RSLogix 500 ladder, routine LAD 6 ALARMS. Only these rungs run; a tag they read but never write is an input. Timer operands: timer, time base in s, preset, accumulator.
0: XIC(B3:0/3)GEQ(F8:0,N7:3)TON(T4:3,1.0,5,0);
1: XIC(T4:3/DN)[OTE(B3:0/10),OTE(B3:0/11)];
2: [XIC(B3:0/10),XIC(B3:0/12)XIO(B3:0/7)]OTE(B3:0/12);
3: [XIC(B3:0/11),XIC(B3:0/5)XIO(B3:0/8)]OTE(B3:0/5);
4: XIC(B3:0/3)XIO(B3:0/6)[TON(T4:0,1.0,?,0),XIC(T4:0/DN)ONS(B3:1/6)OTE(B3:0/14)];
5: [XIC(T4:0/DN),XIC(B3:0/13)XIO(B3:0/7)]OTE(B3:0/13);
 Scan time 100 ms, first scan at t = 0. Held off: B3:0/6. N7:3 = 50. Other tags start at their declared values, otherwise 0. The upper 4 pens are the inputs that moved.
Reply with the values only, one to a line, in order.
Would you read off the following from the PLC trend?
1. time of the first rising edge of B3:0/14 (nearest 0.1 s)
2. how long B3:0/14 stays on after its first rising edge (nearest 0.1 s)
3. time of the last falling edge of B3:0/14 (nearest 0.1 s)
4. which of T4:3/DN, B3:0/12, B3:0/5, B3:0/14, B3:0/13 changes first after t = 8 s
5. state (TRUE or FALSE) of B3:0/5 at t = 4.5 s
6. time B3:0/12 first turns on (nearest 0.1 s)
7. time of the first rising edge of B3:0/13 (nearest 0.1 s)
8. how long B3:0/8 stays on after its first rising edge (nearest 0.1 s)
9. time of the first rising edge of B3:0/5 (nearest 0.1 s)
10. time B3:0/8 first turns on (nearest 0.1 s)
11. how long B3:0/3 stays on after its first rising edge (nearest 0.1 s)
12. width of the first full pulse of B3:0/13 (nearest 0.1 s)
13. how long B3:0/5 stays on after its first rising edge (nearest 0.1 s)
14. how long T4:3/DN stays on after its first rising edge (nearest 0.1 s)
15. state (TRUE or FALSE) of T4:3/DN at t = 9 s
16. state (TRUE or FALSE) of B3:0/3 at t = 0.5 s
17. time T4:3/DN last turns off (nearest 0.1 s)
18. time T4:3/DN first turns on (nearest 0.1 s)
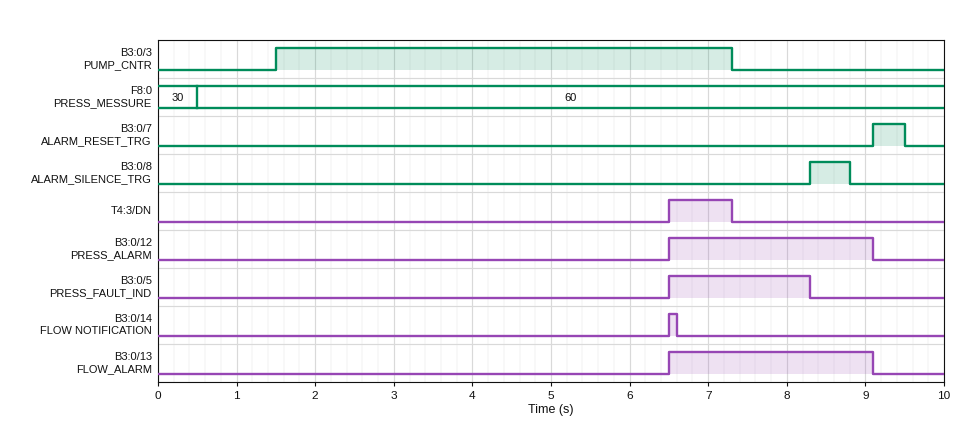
6.5 s
0.1 s
6.6 s
B3:0/5
FALSE
6.5 s
6.5 s
0.5 s
6.5 s
8.3 s
5.8 s
2.6 s
1.8 s
0.8 s
FALSE
FALSE
7.3 s
6.5 s
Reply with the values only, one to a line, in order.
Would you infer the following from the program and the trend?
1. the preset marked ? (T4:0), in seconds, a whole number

5 s
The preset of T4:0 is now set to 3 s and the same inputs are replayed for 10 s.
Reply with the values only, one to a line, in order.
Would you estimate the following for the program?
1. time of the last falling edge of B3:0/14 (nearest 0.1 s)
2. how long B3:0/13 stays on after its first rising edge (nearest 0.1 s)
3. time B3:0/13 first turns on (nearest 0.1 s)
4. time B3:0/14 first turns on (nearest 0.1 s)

4.6 s
4.6 s
4.5 s
4.5 s
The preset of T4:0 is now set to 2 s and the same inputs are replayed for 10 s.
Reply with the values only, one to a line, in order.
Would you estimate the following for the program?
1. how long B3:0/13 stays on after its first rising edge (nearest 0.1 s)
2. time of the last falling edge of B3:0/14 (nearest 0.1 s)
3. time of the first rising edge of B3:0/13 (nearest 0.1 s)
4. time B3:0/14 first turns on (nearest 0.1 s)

5.6 s
3.6 s
3.5 s
3.5 s
